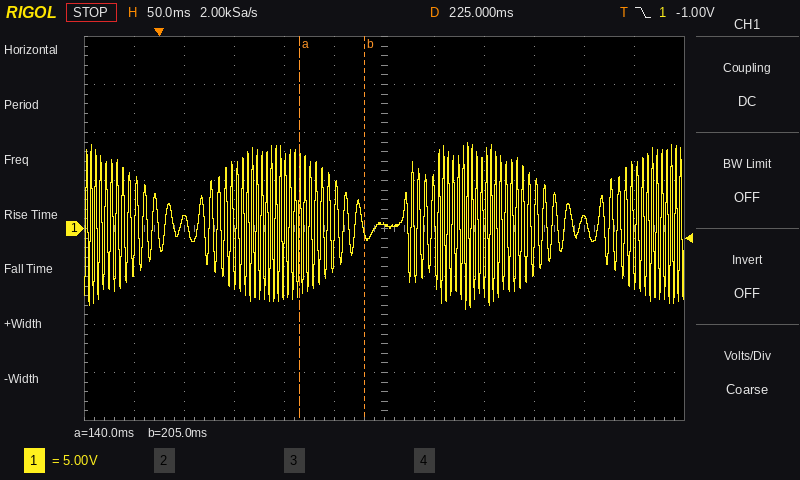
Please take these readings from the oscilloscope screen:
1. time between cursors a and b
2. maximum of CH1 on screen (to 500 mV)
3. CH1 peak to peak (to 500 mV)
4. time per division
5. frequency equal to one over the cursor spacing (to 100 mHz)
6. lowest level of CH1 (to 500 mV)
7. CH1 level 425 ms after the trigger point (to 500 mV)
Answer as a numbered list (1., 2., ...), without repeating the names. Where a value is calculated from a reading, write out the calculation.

1. 205 ms − (140 ms) = 65 ms
2. 9.0 V
3. 9.0 V − (-8.5 V) = 17.5 V
4. 50 ms
5. 1 / 65 ms ≈ 15.4 Hz
6. -8.5 V
7. 1.0 V
